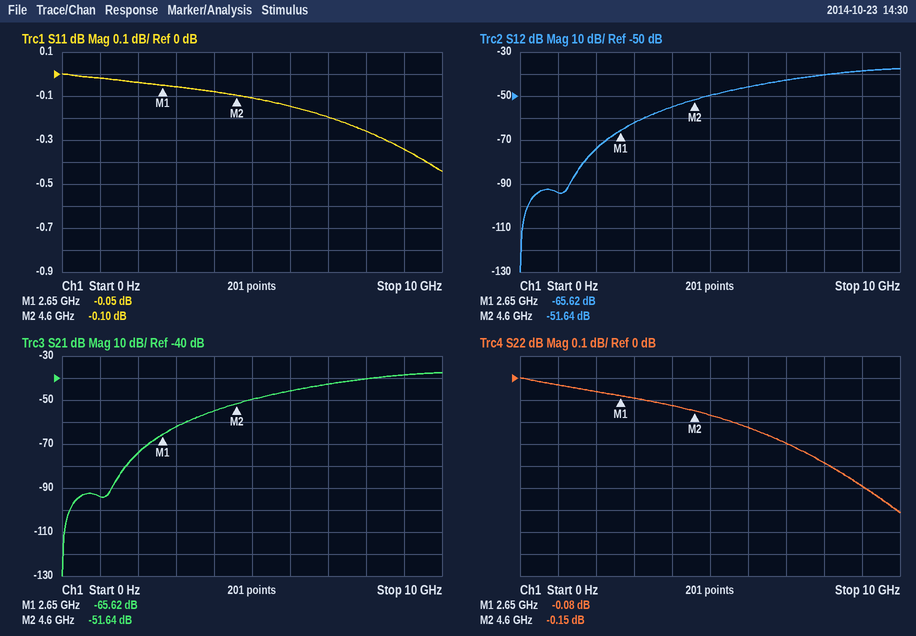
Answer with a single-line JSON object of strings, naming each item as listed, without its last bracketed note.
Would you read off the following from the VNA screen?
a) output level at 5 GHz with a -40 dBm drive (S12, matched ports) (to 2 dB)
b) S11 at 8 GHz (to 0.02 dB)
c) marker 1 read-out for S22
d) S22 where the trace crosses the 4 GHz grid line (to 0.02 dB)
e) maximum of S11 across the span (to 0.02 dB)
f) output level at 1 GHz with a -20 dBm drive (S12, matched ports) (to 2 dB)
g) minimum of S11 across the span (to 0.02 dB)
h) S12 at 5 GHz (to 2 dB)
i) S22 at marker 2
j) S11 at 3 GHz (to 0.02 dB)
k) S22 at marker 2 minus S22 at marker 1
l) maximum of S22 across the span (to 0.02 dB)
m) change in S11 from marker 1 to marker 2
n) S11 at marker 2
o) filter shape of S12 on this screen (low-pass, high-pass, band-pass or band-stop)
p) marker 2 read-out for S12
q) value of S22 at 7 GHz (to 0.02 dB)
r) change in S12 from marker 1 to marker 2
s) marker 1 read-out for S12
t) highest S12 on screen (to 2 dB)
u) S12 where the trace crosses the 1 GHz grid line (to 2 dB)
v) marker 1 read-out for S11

{"output level at 5 GHz with a -40 dBm drive (S12, matched ports)": "-90 dBm", "S11 at 8 GHz": "-0.26 dB", "marker 1 read-out for S22": "-0.08 dB", "S22 where the trace crosses the 4 GHz grid line": "-0.12 dB", "maximum of S11 across the span": "0.00 dB", "output level at 1 GHz with a -20 dBm drive (S12, matched ports)": "-114 dBm", "minimum of S11 across the span": "-0.44 dB", "S12 at 5 GHz": "-50 dB", "S22 at marker 2": "-0.15 dB", "S11 at 3 GHz": "-0.06 dB", "S22 at marker 2 minus S22 at marker 1": "-0.07 dB", "maximum of S22 across the span": "0.00 dB", "change in S11 from marker 1 to marker 2": "-0.05 dB", "S11 at marker 2": "-0.10 dB", "filter shape of S12 on this screen": "high-pass", "marker 2 read-out for S12": "-51.64 dB", "value of S22 at 7 GHz": "-0.30 dB", "change in S12 from marker 1 to marker 2": "13.98 dB", "marker 1 read-out for S12": "-65.62 dB", "highest S12 on screen": "-38 dB", "S12 where the trace crosses the 1 GHz grid line": "-94 dB", "marker 1 read-out for S11": "-0.05 dB"}
